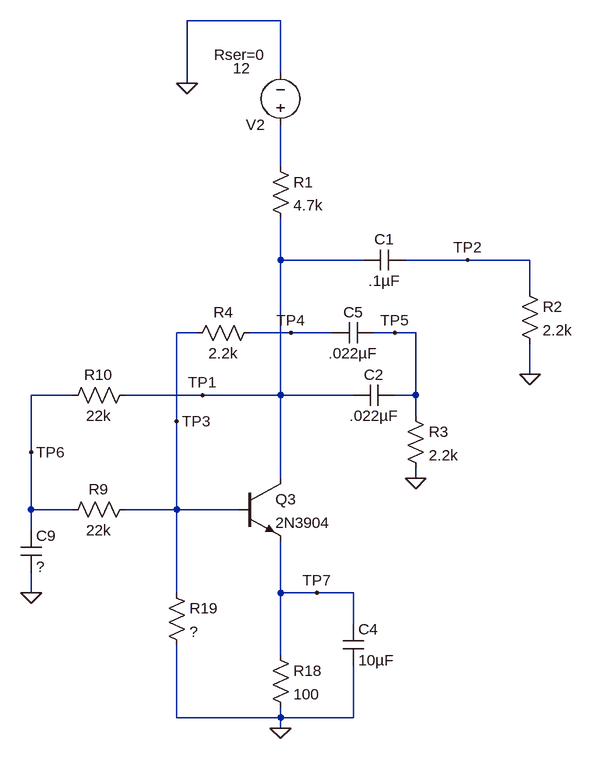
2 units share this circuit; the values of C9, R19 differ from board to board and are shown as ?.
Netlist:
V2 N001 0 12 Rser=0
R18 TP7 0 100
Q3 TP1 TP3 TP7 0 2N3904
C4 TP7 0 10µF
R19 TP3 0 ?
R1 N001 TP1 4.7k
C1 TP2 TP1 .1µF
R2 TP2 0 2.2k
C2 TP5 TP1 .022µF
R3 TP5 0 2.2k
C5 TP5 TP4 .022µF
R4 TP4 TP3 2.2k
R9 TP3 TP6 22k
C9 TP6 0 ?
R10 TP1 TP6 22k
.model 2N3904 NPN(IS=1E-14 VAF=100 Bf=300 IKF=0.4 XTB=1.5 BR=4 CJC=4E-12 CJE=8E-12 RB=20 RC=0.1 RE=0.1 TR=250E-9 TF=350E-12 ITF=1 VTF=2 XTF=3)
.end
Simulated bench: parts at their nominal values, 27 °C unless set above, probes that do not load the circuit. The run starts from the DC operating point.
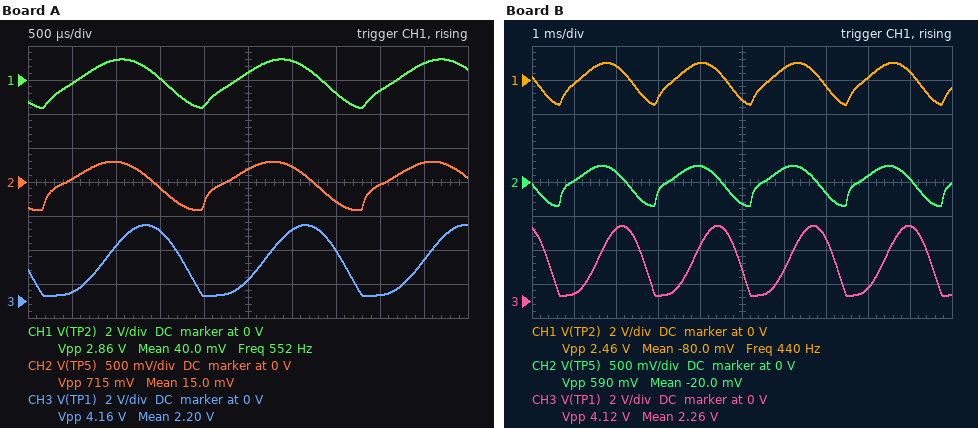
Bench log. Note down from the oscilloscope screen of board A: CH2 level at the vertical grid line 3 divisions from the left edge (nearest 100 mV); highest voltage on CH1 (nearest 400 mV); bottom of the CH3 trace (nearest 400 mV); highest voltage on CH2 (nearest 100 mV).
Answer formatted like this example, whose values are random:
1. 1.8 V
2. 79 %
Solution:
1. -100 mV
2. 1.2 V
3. 400 mV
4. 300 mV
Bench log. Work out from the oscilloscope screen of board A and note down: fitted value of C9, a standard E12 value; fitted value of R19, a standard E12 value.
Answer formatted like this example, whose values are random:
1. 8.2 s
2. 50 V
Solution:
1. 56 nF
2. 39 kΩ
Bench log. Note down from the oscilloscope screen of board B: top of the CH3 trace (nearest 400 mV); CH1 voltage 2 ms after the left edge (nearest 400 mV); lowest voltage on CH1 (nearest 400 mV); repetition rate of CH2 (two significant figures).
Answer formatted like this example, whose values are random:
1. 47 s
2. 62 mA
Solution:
1. 4.4 V
2. 800 mV
3. -1.6 V
4. 440 Hz
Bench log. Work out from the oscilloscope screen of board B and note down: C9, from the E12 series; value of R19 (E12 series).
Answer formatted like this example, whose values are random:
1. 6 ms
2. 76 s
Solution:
1. 120 nF
2. 39 kΩ
